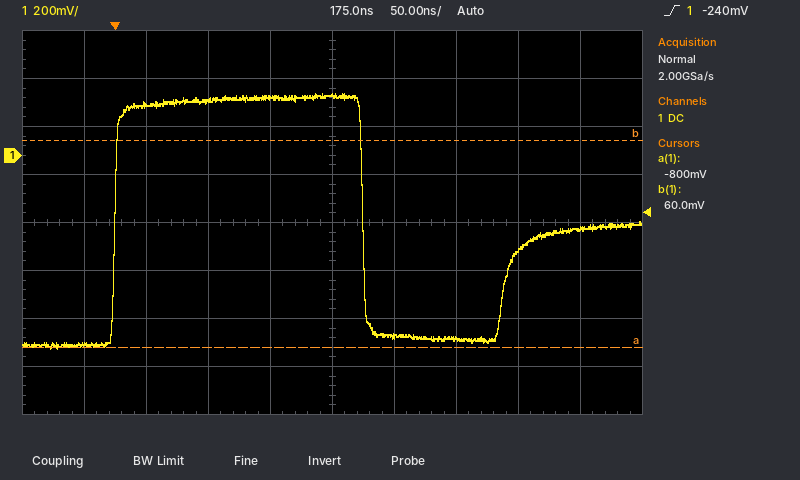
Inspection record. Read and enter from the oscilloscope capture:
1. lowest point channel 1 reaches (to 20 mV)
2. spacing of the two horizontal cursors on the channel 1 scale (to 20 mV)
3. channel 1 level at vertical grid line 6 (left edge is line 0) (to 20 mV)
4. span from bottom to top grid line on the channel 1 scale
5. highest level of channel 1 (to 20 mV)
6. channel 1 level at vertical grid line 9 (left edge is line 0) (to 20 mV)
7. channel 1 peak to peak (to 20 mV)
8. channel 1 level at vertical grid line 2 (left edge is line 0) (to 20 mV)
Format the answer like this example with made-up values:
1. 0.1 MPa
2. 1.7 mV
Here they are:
1. -800 mV
2. 860 mV
3. -760 mV
4. 1.6 V
5. 260 mV
6. -300 mV
7. 1.06 V
8. 220 mV
